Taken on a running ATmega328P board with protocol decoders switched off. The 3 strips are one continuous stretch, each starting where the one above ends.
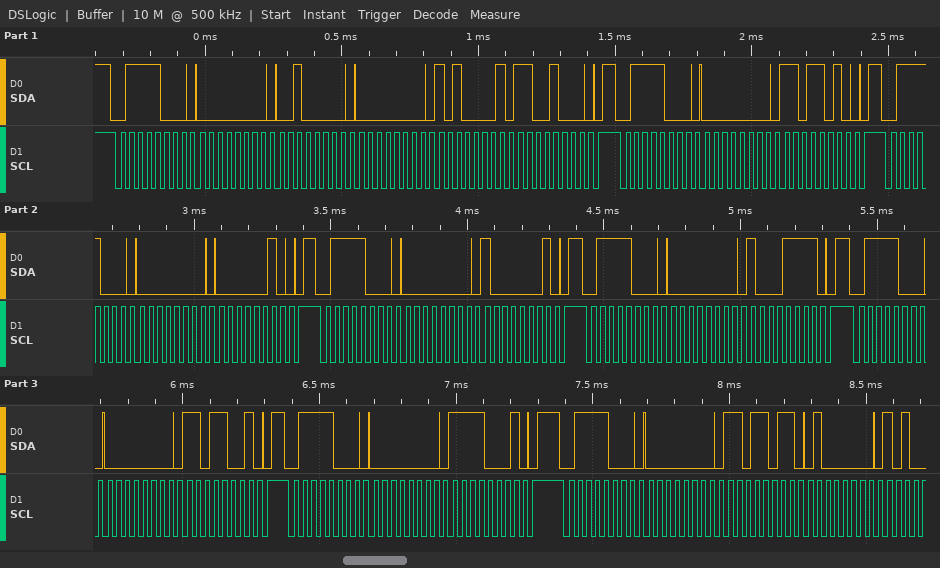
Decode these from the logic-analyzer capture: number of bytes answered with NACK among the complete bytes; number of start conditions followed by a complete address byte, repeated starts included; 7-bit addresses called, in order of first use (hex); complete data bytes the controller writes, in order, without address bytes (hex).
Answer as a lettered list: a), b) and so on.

a) 0
b) 8
c) 0x3C
d) 00 20 00 A1 C8 00 DA 00 02 00 81 00 8F 00 D9 00 F1 00 DB 40
